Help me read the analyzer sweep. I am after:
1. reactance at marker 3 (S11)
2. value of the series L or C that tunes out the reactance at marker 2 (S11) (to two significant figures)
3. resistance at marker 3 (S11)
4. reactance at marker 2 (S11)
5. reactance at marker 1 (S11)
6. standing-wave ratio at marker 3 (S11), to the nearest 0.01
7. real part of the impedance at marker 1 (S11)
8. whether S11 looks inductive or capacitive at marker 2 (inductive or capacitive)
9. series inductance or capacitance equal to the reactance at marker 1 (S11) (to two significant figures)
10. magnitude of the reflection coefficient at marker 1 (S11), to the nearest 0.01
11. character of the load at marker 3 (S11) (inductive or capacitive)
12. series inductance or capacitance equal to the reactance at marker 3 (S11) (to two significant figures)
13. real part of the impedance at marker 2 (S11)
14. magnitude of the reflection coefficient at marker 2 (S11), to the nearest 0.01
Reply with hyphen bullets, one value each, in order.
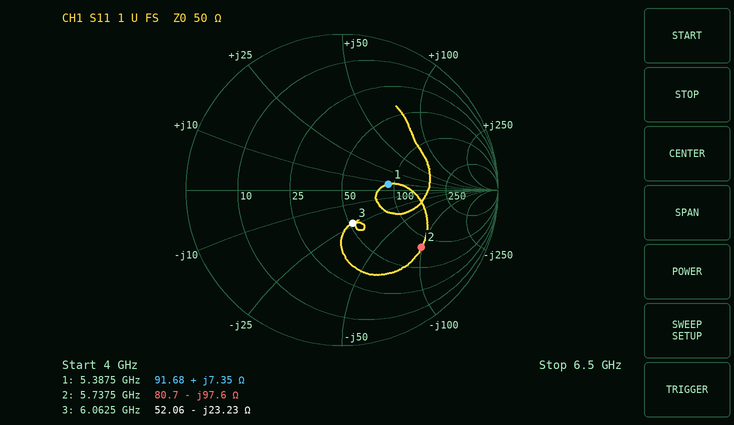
- -23.23 Ω
- 2.7 nH
- 52.06 Ω
- -97.6 Ω
- +7.35 Ω
- 1.57
- 91.68 Ω
- capacitive
- 220 pH
- 0.30
- capacitive
- 1.1 pF
- 80.7 Ω
- 0.63
